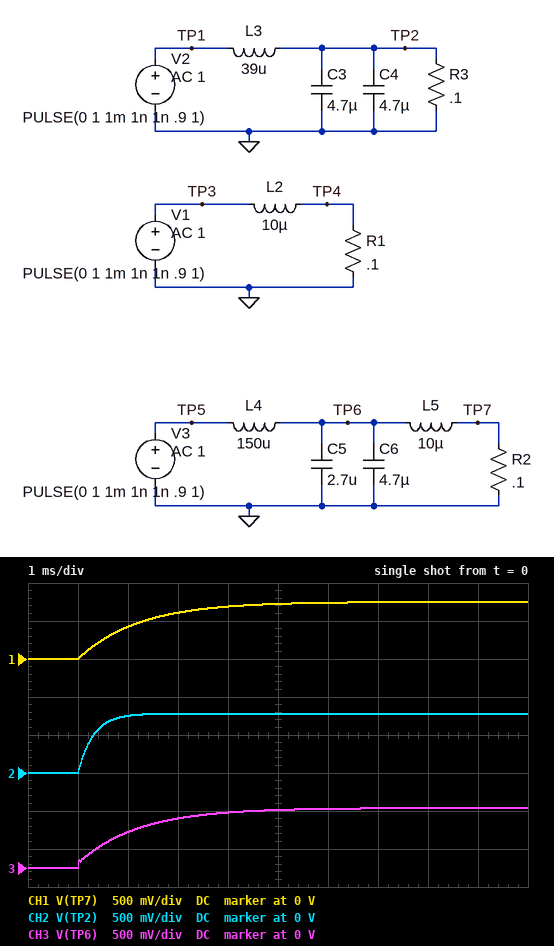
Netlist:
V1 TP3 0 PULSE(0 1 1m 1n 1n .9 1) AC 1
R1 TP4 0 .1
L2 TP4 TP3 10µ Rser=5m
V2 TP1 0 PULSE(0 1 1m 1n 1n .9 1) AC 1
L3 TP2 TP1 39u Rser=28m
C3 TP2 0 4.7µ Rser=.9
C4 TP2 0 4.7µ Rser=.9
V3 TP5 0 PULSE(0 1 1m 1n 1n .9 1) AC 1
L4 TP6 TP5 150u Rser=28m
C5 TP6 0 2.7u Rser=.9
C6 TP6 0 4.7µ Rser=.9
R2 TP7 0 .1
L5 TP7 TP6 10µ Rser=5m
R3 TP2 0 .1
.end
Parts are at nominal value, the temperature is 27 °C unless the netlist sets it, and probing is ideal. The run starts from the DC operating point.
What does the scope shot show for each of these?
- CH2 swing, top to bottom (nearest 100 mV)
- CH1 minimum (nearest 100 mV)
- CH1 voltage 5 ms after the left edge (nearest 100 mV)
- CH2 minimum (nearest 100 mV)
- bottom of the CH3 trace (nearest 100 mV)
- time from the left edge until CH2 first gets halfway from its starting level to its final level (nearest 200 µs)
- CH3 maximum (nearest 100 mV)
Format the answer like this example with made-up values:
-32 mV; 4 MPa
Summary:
800 mV; 0 V; 700 mV; 0 V; 0 V; 1.2 ms; 800 mV
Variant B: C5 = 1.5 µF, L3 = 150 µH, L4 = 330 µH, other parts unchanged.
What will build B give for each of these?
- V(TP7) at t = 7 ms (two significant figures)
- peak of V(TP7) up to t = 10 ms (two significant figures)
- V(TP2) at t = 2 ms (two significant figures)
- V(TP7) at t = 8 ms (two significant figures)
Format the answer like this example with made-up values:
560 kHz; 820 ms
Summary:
680 mV; 730 mV; 450 mV; 700 mV
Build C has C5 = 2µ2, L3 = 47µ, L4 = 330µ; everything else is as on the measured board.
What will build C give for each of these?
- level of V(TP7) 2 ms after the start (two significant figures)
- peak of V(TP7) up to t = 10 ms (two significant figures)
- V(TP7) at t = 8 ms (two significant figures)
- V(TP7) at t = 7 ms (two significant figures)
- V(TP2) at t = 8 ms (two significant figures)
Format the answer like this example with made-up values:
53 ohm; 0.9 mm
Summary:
240 mV; 730 mV; 700 mV; 680 mV; 780 mV
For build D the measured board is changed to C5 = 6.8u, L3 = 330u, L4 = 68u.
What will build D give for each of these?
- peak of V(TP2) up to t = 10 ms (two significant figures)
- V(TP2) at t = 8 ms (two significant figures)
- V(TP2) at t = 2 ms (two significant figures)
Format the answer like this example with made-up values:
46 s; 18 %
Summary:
760 mV; 730 mV; 250 mV
